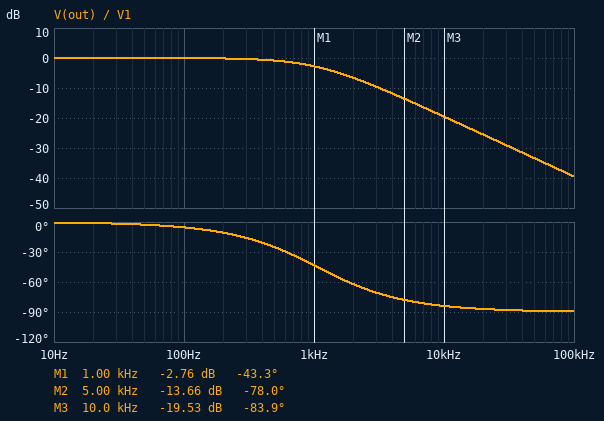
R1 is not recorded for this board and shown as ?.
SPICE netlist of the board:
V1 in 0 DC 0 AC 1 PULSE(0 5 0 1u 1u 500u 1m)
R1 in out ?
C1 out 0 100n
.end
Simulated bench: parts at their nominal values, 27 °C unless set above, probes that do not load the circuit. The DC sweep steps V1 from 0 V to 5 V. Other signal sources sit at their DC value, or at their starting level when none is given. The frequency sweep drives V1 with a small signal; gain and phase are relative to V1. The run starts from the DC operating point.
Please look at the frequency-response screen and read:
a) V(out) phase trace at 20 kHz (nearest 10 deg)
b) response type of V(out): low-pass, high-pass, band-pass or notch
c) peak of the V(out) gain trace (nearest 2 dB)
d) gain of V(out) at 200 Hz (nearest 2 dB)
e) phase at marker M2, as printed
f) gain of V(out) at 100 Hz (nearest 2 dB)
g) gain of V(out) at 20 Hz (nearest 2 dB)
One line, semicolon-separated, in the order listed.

-90 deg; low-pass; 0 dB; 0 dB; -78.0 deg; 0 dB; 0 dB
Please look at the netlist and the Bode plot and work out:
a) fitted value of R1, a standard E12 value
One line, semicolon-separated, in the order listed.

1.5 kΩ
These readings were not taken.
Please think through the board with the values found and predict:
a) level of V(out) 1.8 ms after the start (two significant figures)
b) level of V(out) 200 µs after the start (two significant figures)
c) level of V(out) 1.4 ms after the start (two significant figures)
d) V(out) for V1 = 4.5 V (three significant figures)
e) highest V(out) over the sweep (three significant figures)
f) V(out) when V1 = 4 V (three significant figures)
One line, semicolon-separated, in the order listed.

660 mV; 3.7 V; 4.7 V; 4.50 V; 5.00 V; 4.00 V
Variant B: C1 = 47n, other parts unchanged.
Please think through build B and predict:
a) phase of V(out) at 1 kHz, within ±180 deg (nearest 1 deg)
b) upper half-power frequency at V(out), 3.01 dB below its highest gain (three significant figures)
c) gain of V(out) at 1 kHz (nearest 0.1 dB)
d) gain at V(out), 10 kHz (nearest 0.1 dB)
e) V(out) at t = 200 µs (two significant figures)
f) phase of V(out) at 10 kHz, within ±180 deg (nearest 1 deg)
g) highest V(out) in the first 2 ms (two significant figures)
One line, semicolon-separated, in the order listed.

-24 deg; 2.26 kHz; -0.8 dB; -13.1 dB; 4.7 V; -77 deg; 5.0 V
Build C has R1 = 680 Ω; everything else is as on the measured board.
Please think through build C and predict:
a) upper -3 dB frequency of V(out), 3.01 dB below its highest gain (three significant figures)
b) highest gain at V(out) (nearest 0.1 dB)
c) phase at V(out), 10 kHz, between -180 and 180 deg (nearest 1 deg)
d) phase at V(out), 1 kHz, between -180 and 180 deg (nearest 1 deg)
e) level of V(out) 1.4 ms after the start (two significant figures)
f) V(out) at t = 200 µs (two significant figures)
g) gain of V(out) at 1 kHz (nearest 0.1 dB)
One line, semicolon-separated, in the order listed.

2.34 kHz; 0 dB; -77 deg; -23 deg; 5.0 V; 4.7 V; -0.7 dB
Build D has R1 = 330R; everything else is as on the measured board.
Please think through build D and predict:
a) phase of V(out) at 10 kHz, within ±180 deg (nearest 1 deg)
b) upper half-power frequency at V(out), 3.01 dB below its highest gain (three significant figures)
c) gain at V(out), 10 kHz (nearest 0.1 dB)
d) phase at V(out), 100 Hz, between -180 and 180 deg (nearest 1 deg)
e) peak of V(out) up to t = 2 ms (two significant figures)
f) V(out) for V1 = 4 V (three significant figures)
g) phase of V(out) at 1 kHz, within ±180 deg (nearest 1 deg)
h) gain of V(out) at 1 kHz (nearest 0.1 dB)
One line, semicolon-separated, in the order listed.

-64 deg; 4.82 kHz; -7.2 dB; -1 deg; 5.0 V; 4.00 V; -12 deg; -0.2 dB
